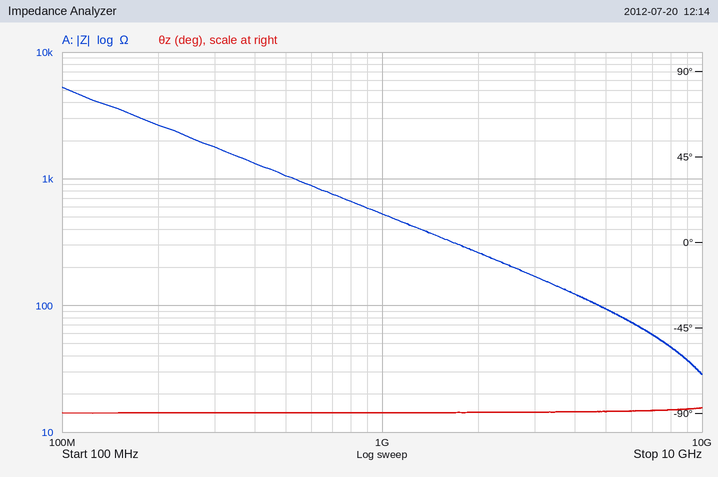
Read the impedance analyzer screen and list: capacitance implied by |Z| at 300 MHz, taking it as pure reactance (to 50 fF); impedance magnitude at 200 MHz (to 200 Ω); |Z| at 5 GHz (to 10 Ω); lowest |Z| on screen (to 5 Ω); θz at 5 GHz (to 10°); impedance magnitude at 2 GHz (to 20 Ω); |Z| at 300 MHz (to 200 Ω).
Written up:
300 fF
2.6 kΩ
90 Ω
30 Ω
-90°
260 Ω
1.8 kΩ
